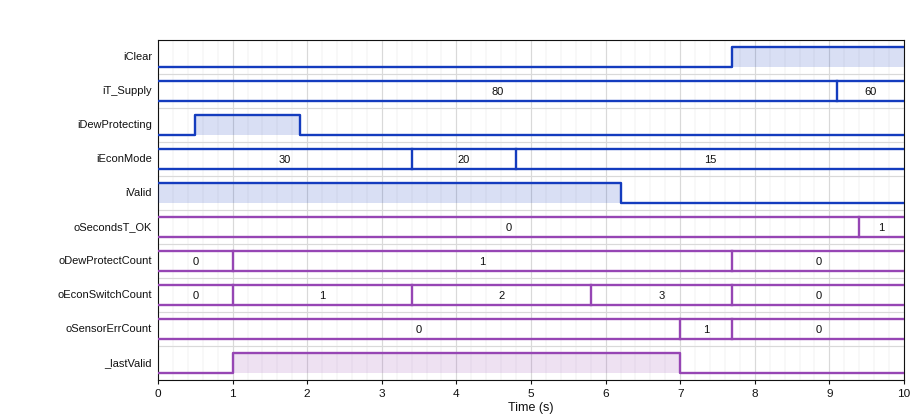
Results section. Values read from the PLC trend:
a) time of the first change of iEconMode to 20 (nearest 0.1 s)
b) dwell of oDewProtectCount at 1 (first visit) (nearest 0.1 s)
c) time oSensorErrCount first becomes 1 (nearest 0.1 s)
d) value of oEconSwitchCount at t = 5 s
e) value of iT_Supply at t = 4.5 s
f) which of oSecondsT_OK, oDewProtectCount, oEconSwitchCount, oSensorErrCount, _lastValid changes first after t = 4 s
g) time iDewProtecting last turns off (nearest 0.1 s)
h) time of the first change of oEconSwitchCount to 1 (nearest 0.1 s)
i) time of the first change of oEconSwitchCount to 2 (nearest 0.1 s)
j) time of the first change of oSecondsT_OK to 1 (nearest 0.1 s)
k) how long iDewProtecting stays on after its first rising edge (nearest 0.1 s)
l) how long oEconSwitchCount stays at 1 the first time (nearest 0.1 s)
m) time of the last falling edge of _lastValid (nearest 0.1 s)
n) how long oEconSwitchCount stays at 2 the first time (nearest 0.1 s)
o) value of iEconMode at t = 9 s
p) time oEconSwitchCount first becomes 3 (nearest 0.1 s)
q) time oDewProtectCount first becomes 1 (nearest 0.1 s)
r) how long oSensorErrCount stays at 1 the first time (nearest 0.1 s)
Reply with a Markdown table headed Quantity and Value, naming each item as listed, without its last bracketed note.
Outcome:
| Quantity | Value |
|---|---|
| time of the first change of iEconMode to 20 | 3.4 s |
| dwell of oDewProtectCount at 1 (first visit) | 6.7 s |
| time oSensorErrCount first becomes 1 | 7.0 s |
| value of oEconSwitchCount at t = 5 s | 2 |
| value of iT_Supply at t = 4.5 s | 80 |
| which of oSecondsT_OK, oDewProtectCount, oEconSwitchCount, oSensorErrCount, _lastValid changes first after t = 4 s | oEconSwitchCount |
| time iDewProtecting last turns off | 1.9 s |
| time of the first change of oEconSwitchCount to 1 | 1.0 s |
| time of the first change of oEconSwitchCount to 2 | 3.4 s |
| time of the first change of oSecondsT_OK to 1 | 9.4 s |
| how long iDewProtecting stays on after its first rising edge | 1.4 s |
| how long oEconSwitchCount stays at 1 the first time | 2.4 s |
| time of the last falling edge of _lastValid | 7.0 s |
| how long oEconSwitchCount stays at 2 the first time | 2.4 s |
| value of iEconMode at t = 9 s | 15 |
| time oEconSwitchCount first becomes 3 | 5.8 s |
| time oDewProtectCount first becomes 1 | 1.0 s |
| how long oSensorErrCount stays at 1 the first time | 0.7 s |
